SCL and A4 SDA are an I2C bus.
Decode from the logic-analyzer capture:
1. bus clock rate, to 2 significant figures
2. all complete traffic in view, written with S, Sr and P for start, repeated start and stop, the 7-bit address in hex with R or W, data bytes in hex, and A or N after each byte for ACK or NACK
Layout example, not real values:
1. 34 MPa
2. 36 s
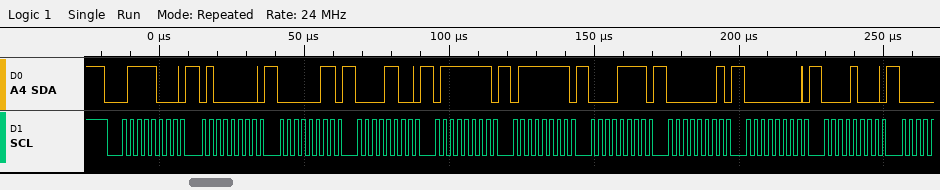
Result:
1. 400 kHz
2. S 3CW A 40 A 03 A 0C A 7F A 7F A 0F A 01 A 00 A 08 A
